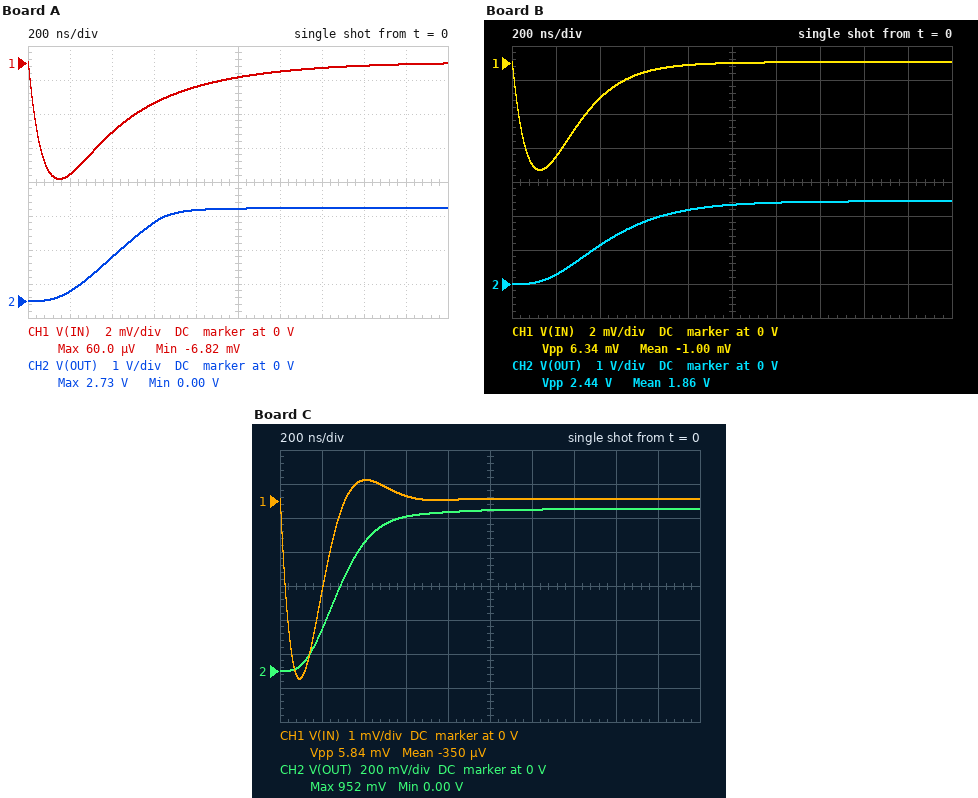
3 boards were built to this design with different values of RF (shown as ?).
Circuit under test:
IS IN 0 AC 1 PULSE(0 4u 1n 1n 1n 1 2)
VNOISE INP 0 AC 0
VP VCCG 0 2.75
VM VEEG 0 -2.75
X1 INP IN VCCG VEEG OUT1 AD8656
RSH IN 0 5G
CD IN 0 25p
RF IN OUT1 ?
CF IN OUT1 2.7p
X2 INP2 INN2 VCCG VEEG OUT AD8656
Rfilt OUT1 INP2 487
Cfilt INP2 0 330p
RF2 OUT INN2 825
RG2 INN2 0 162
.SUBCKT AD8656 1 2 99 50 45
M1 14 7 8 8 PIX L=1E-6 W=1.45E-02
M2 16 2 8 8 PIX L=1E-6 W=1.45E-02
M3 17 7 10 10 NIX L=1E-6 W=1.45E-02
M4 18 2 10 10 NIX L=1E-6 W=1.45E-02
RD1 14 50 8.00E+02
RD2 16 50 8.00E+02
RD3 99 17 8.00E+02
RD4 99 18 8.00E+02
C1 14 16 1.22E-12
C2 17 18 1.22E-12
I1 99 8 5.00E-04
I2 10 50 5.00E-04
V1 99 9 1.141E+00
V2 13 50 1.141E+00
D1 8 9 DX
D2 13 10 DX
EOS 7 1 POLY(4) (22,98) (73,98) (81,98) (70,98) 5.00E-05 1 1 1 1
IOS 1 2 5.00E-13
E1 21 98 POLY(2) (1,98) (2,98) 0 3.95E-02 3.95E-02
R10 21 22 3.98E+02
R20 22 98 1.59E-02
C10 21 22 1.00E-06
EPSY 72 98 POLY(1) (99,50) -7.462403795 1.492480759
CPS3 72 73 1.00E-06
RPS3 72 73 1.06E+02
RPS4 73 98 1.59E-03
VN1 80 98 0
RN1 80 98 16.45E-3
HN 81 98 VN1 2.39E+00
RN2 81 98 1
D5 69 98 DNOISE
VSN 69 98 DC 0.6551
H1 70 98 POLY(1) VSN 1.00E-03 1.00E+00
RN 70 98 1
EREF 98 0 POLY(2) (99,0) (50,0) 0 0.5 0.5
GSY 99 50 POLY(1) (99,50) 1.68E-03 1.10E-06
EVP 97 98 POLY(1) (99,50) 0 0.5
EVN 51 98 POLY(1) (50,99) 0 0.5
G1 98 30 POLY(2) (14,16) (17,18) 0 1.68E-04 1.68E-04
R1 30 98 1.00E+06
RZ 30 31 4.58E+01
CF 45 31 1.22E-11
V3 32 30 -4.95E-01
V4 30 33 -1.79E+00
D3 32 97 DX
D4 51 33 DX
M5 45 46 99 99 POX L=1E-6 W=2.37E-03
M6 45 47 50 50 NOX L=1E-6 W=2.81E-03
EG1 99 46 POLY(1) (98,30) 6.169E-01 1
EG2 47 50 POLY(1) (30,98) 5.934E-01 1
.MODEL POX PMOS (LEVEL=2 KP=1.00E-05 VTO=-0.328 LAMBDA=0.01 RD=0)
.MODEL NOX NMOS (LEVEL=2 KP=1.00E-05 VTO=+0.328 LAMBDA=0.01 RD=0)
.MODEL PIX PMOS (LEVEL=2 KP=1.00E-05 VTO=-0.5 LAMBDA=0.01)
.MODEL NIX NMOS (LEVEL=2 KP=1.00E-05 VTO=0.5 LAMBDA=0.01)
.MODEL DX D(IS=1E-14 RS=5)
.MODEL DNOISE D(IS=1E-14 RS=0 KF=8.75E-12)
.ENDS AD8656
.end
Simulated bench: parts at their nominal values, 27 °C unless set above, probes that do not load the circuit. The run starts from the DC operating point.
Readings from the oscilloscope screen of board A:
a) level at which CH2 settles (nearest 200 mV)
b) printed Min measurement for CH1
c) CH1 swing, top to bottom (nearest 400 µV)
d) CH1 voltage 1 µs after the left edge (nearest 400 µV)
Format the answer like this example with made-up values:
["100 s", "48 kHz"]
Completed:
["2.8 V", "-6.82 mV", "6.8 mV", "-800 µV"]
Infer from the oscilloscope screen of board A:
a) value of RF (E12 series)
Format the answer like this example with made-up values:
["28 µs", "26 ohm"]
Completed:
["180 kΩ"]
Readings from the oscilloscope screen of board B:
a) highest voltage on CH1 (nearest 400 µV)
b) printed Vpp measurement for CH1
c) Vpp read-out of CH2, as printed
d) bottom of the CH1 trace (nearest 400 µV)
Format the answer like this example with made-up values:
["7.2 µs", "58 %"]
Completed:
["0 V", "6.34 mV", "2.44 V", "-6.4 mV"]
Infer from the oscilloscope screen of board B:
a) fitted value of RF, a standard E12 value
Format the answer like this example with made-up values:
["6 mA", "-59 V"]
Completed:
["100 kΩ"]
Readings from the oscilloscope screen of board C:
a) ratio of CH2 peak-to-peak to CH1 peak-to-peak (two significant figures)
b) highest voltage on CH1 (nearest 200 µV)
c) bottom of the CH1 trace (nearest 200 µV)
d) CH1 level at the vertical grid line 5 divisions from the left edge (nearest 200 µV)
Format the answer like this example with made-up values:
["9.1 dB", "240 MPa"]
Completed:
["160", "600 µV", "-5.2 mV", "0 V"]
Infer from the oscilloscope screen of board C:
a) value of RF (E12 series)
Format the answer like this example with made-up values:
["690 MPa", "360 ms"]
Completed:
["39 kΩ"]
